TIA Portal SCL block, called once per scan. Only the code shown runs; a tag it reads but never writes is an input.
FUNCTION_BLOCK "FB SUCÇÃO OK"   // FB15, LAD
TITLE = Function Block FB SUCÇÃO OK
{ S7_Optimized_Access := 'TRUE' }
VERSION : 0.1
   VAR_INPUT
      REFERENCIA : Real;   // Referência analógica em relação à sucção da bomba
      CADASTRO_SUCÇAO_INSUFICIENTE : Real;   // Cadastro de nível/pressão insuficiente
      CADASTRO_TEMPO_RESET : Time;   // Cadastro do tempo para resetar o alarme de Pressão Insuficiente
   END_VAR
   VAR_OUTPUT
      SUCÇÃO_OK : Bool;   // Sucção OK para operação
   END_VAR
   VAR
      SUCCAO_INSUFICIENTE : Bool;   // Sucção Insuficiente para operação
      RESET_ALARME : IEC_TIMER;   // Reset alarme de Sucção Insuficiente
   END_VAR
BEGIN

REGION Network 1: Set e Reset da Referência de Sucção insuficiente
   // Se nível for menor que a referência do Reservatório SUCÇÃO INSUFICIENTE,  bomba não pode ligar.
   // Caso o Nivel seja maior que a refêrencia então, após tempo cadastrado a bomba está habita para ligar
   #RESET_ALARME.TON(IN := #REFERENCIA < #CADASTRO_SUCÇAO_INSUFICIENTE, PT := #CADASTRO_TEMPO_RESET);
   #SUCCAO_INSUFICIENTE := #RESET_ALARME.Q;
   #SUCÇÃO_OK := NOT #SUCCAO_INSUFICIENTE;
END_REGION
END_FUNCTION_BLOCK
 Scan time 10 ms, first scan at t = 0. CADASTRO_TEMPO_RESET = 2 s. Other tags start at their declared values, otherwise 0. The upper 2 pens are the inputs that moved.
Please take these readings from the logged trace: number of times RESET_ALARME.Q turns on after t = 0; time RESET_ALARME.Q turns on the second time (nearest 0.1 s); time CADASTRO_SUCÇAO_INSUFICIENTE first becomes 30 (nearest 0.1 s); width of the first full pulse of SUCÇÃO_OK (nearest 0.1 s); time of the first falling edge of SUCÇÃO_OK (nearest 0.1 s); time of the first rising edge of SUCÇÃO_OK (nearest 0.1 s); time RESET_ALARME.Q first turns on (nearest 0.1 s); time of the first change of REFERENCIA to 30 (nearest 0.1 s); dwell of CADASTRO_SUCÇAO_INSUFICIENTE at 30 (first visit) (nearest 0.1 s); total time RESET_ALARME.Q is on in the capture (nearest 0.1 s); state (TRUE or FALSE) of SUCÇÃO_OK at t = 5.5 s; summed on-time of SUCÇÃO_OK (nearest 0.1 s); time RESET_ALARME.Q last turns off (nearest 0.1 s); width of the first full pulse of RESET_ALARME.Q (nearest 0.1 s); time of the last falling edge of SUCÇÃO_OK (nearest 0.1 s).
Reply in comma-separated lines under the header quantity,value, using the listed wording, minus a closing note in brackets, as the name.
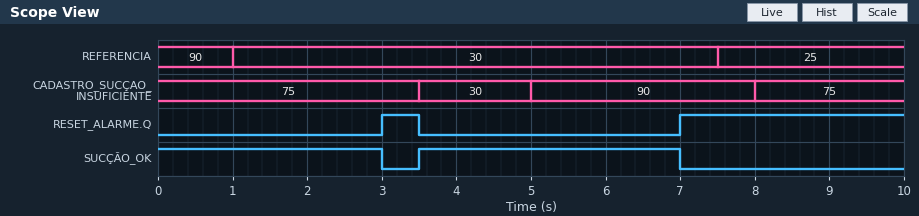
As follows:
quantity,value
number of times RESET_ALARME.Q turns on after t = 0,2
time RESET_ALARME.Q turns on the second time,7.0 s
time CADASTRO_SUCÇAO_INSUFICIENTE first becomes 30,3.5 s
width of the first full pulse of SUCÇÃO_OK,3.5 s
time of the first falling edge of SUCÇÃO_OK,3.0 s
time of the first rising edge of SUCÇÃO_OK,3.5 s
time RESET_ALARME.Q first turns on,3.0 s
time of the first change of REFERENCIA to 30,1.0 s
dwell of CADASTRO_SUCÇAO_INSUFICIENTE at 30 (first visit),1.5 s
total time RESET_ALARME.Q is on in the capture,3.5 s
state (TRUE or FALSE) of SUCÇÃO_OK at t = 5.5 s,TRUE
summed on-time of SUCÇÃO_OK,6.5 s
time RESET_ALARME.Q last turns off,3.5 s
width of the first full pulse of RESET_ALARME.Q,0.5 s
time of the last falling edge of SUCÇÃO_OK,7.0 s
